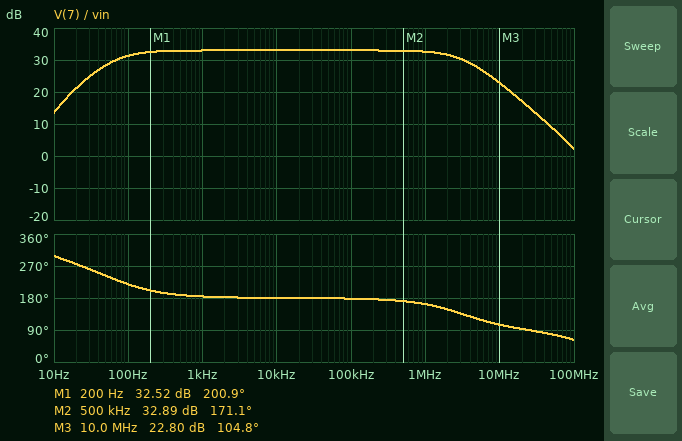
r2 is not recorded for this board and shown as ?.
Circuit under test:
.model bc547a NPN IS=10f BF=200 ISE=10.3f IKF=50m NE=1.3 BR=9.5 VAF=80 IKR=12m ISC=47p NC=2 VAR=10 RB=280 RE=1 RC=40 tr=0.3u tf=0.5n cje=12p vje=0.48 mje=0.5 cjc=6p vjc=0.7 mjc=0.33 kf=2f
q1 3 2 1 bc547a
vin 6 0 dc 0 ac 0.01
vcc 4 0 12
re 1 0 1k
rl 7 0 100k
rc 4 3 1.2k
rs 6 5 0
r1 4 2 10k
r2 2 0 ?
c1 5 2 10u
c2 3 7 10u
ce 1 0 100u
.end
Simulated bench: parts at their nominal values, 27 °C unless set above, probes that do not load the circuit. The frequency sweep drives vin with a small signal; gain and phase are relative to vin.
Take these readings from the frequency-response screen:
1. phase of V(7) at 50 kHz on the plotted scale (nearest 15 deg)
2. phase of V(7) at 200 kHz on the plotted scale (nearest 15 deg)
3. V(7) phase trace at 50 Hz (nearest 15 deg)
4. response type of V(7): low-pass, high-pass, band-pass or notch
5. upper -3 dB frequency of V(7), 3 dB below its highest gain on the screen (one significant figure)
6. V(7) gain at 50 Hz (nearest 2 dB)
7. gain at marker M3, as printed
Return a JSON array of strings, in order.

["180 deg", "180 deg", "240 deg", "band-pass", "3 MHz", "28 dB", "22.80 dB"]
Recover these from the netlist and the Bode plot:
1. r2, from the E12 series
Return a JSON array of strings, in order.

["1.8 kΩ"]
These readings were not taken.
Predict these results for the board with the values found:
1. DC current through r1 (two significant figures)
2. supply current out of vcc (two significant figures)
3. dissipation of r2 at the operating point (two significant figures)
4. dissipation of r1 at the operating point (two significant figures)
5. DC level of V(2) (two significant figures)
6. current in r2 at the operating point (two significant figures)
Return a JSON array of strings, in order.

["1.0 mA", "2.2 mA", "1.8 mW", "10 mW", "1.8 V", "1.0 mA"]
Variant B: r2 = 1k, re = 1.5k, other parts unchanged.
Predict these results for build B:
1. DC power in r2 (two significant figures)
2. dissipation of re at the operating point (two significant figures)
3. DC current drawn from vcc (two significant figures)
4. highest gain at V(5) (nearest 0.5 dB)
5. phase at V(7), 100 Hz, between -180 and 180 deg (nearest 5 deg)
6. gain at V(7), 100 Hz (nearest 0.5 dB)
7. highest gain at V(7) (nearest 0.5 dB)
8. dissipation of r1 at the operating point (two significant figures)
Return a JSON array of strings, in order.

["1.2 mW", "140 µW", "1.4 mA", "0 dB", "-160 deg", "22.0 dB", "22.5 dB", "12 mW"]
